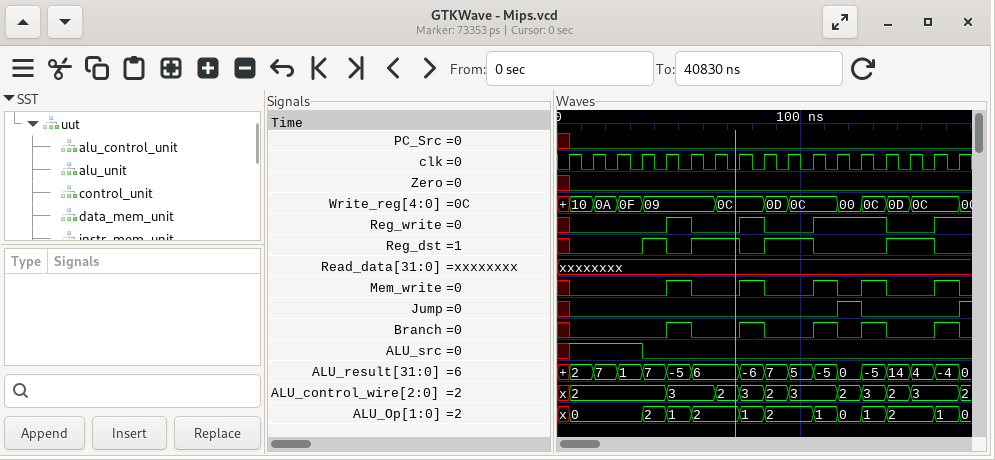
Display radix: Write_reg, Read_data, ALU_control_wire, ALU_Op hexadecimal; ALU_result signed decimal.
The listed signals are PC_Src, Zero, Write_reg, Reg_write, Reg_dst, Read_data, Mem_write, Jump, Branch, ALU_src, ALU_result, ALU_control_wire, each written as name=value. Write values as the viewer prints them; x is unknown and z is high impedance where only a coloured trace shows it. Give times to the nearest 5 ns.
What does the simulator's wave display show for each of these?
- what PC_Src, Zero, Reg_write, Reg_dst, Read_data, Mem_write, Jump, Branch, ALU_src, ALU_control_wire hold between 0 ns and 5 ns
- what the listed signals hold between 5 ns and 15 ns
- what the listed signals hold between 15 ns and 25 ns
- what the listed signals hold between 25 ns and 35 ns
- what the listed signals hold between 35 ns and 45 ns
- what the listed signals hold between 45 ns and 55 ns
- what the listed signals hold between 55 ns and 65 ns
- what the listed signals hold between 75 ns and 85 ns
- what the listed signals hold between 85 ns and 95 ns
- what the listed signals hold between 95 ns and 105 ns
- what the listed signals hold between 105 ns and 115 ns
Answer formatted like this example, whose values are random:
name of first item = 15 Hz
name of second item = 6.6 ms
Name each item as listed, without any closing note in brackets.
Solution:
what PC_Src, Zero, Reg_write, Reg_dst, Read_data, Mem_write, Jump, Branch, ALU_src, ALU_control_wire hold between 0 ns and 5 ns = PC_Src=x, Zero=x, Reg_write=x, Reg_dst=x, Read_data=xxxxxxxx, Mem_write=x, Jump=x, Branch=x, ALU_src=x, ALU_control_wire=x
what the listed signals hold between 5 ns and 15 ns = PC_Src=0, Zero=0, Write_reg=10, Reg_write=0, Reg_dst=0, Read_data=xxxxxxxx, Mem_write=0, Jump=0, Branch=0, ALU_src=1, ALU_result=2, ALU_control_wire=2
what the listed signals hold between 15 ns and 25 ns = PC_Src=0, Zero=0, Write_reg=0A, Reg_write=0, Reg_dst=0, Read_data=xxxxxxxx, Mem_write=0, Jump=0, Branch=0, ALU_src=1, ALU_result=7, ALU_control_wire=2
what the listed signals hold between 25 ns and 35 ns = PC_Src=0, Zero=0, Write_reg=0F, Reg_write=0, Reg_dst=0, Read_data=xxxxxxxx, Mem_write=0, Jump=0, Branch=0, ALU_src=1, ALU_result=1, ALU_control_wire=2
what the listed signals hold between 35 ns and 45 ns = PC_Src=0, Zero=0, Write_reg=09, Reg_write=0, Reg_dst=1, Read_data=xxxxxxxx, Mem_write=0, Jump=0, Branch=0, ALU_src=0, ALU_result=7, ALU_control_wire=2
what the listed signals hold between 45 ns and 55 ns = PC_Src=0, Zero=0, Write_reg=09, Reg_write=1, Reg_dst=0, Read_data=xxxxxxxx, Mem_write=1, Jump=0, Branch=1, ALU_src=0, ALU_result=-5, ALU_control_wire=3
what the listed signals hold between 55 ns and 65 ns = PC_Src=0, Zero=0, Write_reg=09, Reg_write=0, Reg_dst=1, Read_data=xxxxxxxx, Mem_write=0, Jump=0, Branch=0, ALU_src=0, ALU_result=6, ALU_control_wire=3
what the listed signals hold between 75 ns and 85 ns = PC_Src=0, Zero=0, Write_reg=0C, Reg_write=1, Reg_dst=0, Read_data=xxxxxxxx, Mem_write=1, Jump=0, Branch=1, ALU_src=0, ALU_result=-6, ALU_control_wire=3
what the listed signals hold between 85 ns and 95 ns = PC_Src=0, Zero=0, Write_reg=0D, Reg_write=0, Reg_dst=1, Read_data=xxxxxxxx, Mem_write=0, Jump=0, Branch=0, ALU_src=0, ALU_result=7, ALU_control_wire=2
what the listed signals hold between 95 ns and 105 ns = PC_Src=0, Zero=0, Write_reg=0C, Reg_write=0, Reg_dst=1, Read_data=xxxxxxxx, Mem_write=0, Jump=0, Branch=0, ALU_src=0, ALU_result=5, ALU_control_wire=3
what the listed signals hold between 105 ns and 115 ns = PC_Src=0, Zero=0, Write_reg=0C, Reg_write=1, Reg_dst=0, Read_data=xxxxxxxx, Mem_write=1, Jump=0, Branch=1, ALU_src=0, ALU_result=-5, ALU_control_wire=3
